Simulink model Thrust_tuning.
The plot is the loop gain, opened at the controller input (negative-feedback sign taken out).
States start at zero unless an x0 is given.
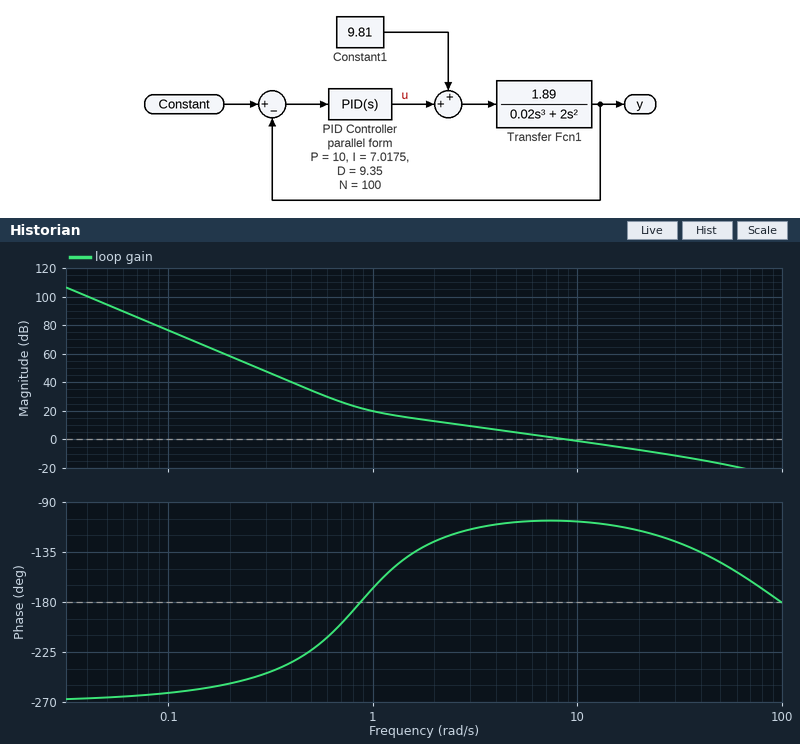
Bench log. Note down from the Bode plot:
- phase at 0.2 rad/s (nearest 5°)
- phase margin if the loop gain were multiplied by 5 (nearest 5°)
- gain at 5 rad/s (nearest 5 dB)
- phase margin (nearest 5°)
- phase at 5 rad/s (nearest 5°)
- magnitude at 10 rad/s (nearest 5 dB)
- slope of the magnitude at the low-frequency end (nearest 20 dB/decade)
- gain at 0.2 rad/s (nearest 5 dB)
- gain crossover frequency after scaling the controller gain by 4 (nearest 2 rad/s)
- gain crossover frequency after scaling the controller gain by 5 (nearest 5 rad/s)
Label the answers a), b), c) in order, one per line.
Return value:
a) -255°
b) 45°
c) 5 dB
d) 75°
e) -110°
f) 0 dB
g) -60 dB/decade
h) 60 dB
i) 32 rad/s
j) 40 rad/s
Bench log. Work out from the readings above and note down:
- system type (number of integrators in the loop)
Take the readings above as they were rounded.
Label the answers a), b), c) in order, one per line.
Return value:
a) 3
